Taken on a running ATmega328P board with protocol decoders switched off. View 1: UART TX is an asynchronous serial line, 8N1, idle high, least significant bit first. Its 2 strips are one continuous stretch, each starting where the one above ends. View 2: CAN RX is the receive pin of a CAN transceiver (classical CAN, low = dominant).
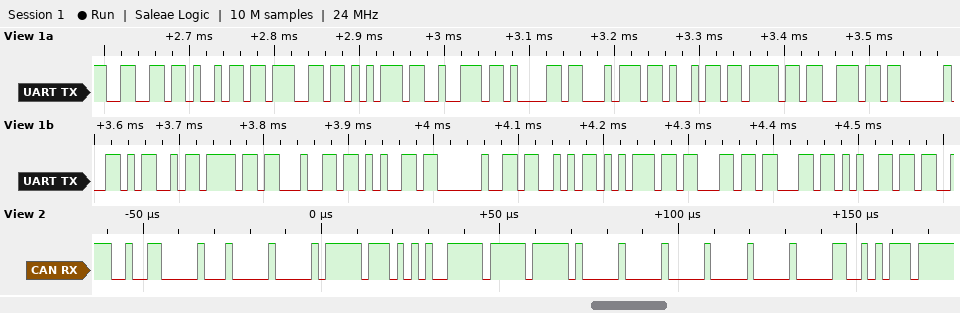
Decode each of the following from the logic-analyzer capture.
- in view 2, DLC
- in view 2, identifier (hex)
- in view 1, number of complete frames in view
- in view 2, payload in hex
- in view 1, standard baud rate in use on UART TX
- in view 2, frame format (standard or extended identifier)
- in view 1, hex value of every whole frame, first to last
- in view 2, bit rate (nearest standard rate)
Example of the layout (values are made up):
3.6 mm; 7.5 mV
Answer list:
8; 0x260; 21; 00 FF 54 FF FF 00 00 00; 115200 baud; standard; 66 69 67 75 72 61 74 69 6F 6E 20 4D 6F 64 65 20 53 75 63 63 65; 500 kbit/s
